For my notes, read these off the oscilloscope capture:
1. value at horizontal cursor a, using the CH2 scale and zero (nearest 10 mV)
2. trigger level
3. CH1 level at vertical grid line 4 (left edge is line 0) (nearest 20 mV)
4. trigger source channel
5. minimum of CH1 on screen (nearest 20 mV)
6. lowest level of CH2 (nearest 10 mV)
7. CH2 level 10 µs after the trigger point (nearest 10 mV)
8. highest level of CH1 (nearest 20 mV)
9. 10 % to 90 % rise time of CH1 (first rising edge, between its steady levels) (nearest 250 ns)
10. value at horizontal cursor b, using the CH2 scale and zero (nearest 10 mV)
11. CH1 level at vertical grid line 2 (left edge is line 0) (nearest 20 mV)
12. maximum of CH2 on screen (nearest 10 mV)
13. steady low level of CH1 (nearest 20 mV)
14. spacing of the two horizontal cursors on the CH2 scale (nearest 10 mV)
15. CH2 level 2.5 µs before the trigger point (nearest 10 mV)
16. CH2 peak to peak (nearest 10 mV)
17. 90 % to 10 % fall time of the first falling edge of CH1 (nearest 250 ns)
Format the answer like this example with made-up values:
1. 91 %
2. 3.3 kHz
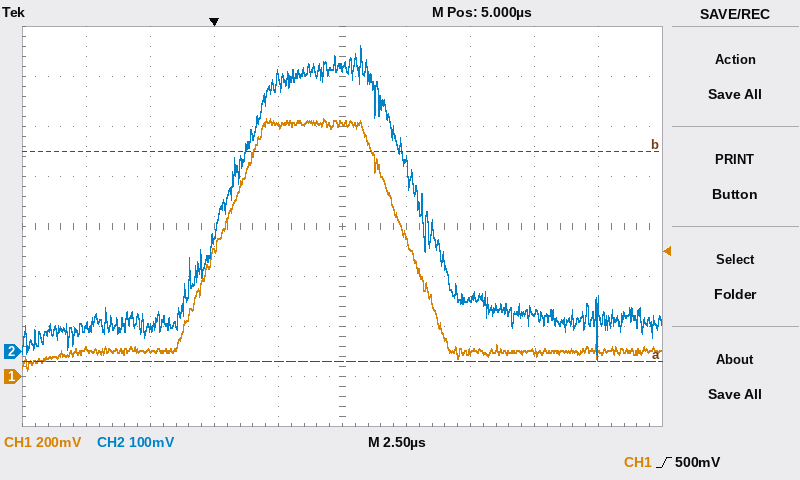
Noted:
1. -20 mV
2. 500 mV
3. 1.00 V
4. CH1
5. 20 mV
6. -20 mV
7. 110 mV
8. 1.04 V
9. 2.75 µs
10. 400 mV
11. 100 mV
12. 610 mV
13. 100 mV
14. 420 mV
15. 50 mV
16. 630 mV
17. 2.75 µs
